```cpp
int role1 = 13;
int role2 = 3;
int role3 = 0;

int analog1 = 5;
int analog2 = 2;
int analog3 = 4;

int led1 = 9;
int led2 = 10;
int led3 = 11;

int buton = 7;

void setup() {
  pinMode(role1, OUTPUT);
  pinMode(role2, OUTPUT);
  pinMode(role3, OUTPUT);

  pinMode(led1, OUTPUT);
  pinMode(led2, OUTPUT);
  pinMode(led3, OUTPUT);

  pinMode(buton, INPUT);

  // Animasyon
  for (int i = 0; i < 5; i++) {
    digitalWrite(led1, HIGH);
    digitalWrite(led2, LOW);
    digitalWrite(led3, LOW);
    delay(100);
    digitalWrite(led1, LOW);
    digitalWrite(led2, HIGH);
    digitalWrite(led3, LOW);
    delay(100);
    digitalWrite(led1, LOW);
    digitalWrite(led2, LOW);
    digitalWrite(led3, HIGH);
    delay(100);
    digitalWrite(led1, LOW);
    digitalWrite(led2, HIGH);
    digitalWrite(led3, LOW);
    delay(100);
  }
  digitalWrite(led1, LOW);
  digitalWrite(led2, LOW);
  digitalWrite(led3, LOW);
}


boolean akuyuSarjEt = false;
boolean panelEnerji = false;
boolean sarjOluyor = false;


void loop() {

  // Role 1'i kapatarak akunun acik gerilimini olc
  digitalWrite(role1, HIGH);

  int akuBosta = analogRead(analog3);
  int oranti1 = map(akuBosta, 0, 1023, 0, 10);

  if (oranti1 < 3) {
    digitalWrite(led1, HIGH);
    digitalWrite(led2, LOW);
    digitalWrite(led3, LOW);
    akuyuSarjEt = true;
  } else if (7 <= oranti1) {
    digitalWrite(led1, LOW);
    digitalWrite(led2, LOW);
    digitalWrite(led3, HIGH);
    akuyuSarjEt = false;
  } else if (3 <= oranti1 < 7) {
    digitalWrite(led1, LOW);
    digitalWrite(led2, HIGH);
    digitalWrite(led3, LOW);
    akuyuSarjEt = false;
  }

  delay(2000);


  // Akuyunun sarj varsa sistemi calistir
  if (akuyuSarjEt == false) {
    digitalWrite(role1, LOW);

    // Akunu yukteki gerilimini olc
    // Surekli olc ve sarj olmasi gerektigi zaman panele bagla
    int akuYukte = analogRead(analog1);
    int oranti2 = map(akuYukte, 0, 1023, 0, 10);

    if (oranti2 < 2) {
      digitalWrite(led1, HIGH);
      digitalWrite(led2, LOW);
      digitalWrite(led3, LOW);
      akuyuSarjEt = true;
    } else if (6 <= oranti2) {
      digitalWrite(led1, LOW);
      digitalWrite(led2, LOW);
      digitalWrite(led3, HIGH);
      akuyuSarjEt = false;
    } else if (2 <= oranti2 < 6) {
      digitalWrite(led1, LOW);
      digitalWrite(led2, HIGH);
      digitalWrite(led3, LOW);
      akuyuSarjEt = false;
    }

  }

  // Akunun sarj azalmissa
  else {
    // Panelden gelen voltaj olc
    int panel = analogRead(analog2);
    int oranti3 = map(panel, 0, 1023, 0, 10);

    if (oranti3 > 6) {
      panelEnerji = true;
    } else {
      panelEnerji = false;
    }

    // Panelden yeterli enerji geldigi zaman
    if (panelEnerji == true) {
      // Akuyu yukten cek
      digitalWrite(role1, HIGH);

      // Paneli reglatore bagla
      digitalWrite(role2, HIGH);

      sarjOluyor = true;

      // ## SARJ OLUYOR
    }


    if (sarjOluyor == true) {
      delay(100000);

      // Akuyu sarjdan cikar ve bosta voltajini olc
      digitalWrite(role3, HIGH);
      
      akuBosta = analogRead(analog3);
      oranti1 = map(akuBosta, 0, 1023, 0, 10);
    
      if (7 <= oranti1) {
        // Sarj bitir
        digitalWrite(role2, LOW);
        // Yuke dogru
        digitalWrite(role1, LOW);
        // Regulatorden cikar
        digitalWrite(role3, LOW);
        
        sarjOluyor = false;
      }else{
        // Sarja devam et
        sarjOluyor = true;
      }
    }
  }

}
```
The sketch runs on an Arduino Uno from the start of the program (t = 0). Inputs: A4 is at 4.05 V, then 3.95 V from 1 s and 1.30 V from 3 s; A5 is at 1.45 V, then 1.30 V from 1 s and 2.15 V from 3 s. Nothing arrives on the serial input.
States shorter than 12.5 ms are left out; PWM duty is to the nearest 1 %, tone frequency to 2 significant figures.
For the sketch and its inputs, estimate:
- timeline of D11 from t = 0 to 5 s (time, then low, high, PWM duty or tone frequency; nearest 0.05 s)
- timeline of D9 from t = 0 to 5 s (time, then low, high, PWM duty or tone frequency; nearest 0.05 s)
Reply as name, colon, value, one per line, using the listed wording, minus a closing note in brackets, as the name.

timeline of D11 from t = 0 to 5 s: 0 s low; 0.2 s high; 0.3 s low; 0.6 s high; 0.7 s low; 1 s high; 1.1 s low; 1.4 s high; 1.5 s low; 1.8 s high; 1.9 s low; 2 s high; 4 s low
timeline of D9 from t = 0 to 5 s: 0 s high; 0.1 s low; 0.4 s high; 0.5 s low; 0.8 s high; 0.9 s low; 1.2 s high; 1.3 s low; 1.6 s high; 1.7 s low; 4 s high
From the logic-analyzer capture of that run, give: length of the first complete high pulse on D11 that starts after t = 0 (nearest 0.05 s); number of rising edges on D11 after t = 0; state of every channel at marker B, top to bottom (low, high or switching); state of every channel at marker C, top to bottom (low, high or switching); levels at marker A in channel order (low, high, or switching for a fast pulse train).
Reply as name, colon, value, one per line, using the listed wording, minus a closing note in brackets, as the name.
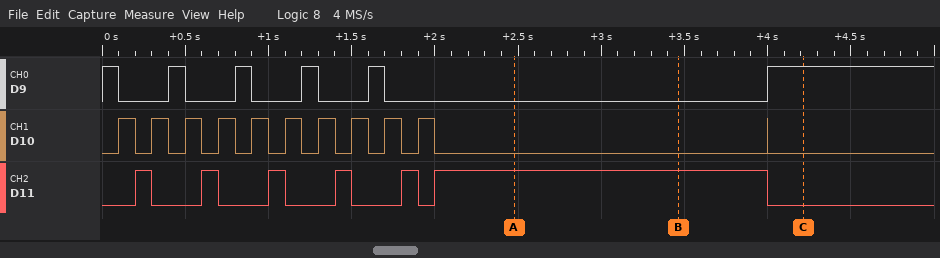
length of the first complete high pulse on D11 that starts after t = 0: 0.10 s
number of rising edges on D11 after t = 0: 6
state of every channel at marker B, top to bottom: D9 low, D10 low, D11 high
state of every channel at marker C, top to bottom: D9 high, D10 low, D11 low
levels at marker A in channel order: D9 low, D10 low, D11 high
